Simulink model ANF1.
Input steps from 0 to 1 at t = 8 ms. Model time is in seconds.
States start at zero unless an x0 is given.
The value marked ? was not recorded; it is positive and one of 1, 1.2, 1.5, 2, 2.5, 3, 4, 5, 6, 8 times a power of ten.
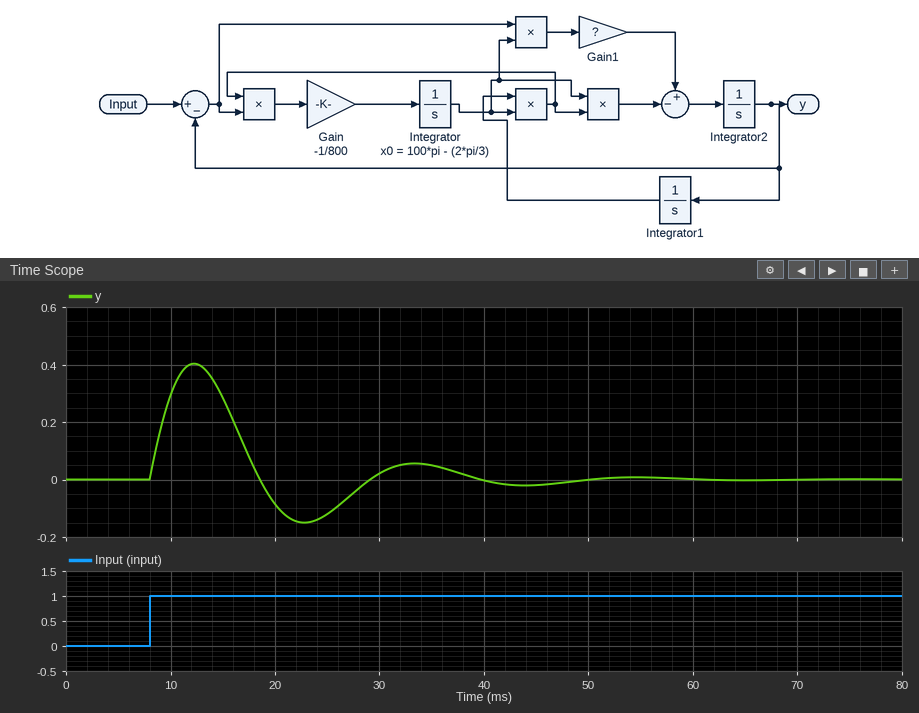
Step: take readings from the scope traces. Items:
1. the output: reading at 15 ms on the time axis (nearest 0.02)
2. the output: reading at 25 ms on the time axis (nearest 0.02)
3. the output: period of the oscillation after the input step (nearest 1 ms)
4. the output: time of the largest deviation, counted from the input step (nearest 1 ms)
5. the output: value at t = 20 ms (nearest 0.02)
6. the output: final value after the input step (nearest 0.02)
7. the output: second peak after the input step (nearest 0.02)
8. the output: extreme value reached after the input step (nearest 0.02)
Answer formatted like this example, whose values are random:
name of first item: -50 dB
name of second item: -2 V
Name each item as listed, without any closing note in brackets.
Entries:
the output: reading at 15 ms on the time axis: 0.28
the output: reading at 25 ms on the time axis: -0.12
the output: period of the oscillation after the input step: 21 ms
the output: time of the largest deviation, counted from the input step: 4 ms
the output: value at t = 20 ms: -0.08
the output: final value after the input step: 0.00
the output: second peak after the input step: 0.06
the output: extreme value reached after the input step: 0.40
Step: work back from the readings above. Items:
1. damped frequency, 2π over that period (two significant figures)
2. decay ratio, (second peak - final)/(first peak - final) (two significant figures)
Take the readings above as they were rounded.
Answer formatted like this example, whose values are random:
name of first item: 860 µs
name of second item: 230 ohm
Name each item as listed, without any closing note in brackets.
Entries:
damped frequency, 2π over that period: 0.30 rad/ms
decay ratio, (second peak - final)/(first peak - final): 0.15
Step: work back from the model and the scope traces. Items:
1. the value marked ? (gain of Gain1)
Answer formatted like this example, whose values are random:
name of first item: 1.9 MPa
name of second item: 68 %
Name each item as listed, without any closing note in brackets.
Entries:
the value marked ?: 0.6
